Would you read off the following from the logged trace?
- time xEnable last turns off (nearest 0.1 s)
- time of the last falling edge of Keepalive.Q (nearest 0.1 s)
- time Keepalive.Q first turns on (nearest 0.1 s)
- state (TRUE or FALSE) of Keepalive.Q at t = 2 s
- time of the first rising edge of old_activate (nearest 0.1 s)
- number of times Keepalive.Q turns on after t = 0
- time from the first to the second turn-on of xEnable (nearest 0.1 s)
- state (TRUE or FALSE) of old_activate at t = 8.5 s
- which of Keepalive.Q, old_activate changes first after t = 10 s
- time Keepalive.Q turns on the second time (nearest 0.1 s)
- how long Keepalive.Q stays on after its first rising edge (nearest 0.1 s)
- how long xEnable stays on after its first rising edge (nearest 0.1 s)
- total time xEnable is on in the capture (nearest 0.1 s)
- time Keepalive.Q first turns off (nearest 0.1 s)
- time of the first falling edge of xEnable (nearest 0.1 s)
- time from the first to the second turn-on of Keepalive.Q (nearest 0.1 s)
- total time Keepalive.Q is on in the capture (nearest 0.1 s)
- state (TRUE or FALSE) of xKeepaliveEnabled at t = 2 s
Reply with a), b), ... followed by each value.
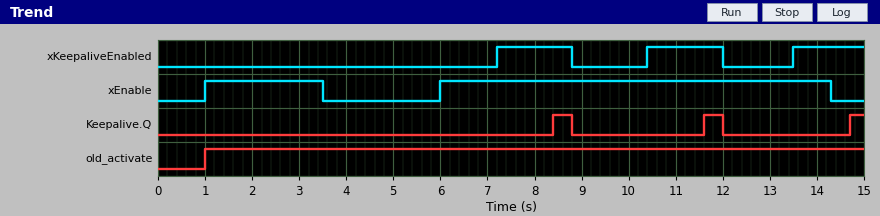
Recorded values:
a) 14.3 s
b) 12.0 s
c) 8.4 s
d) FALSE
e) 1.0 s
f) 3
g) 5.0 s
h) TRUE
i) Keepalive.Q
j) 11.6 s
k) 0.4 s
l) 2.5 s
m) 10.8 s
n) 8.8 s
o) 3.5 s
p) 3.2 s
q) 1.1 s
r) FALSE
